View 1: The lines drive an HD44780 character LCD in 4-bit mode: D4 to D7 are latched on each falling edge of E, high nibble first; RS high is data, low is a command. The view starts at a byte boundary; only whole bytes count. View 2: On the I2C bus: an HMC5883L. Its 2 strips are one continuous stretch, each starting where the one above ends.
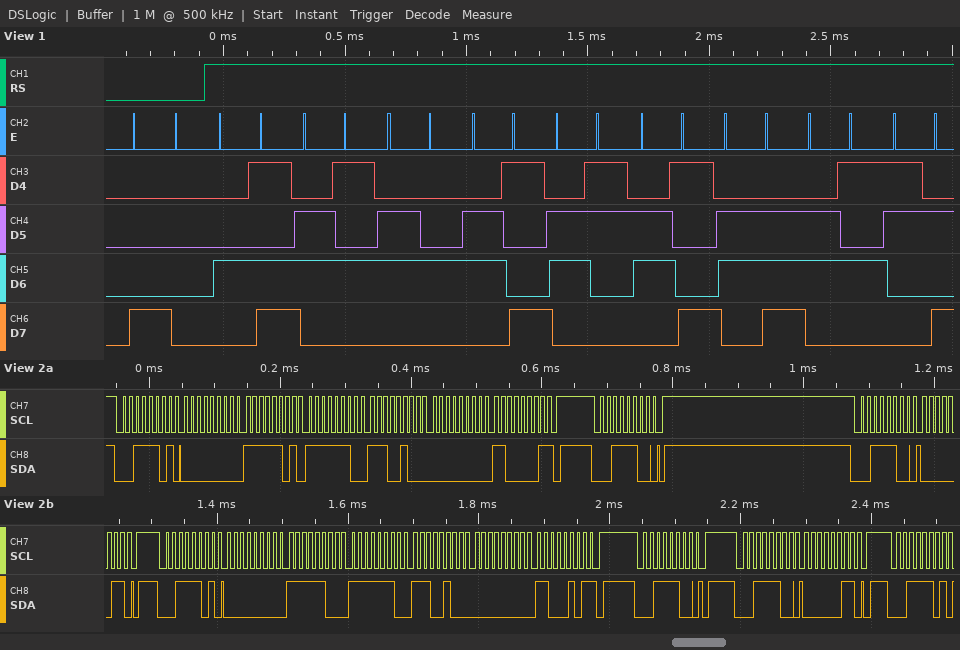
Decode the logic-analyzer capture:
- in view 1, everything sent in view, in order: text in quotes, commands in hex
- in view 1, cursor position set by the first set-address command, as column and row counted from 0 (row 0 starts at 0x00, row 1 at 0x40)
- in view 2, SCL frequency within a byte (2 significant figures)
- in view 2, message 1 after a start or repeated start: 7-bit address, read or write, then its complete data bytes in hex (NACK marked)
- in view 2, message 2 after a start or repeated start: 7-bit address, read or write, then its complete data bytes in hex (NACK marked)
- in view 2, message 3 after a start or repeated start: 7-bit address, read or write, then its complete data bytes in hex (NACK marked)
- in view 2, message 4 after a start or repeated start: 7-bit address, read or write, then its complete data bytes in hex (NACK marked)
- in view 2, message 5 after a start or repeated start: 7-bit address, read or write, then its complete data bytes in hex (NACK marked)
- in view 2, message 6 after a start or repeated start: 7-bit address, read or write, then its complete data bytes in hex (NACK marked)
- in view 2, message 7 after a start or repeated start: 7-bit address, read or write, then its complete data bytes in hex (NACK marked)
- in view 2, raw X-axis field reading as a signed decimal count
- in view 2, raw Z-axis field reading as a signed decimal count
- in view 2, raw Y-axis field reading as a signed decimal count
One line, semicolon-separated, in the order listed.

0x80 "Medicine:"; column 0, row 0; 100 kHz; 0x1E read: 00 FD FE E4 00 C1 NACK; 0x1E write; 0x1E write: 03; 0x1E read: 00 FC FE E4 00 C5 NACK; 0x1E write; 0x1E write: 03; 0x1E read; 252; -284; 197
